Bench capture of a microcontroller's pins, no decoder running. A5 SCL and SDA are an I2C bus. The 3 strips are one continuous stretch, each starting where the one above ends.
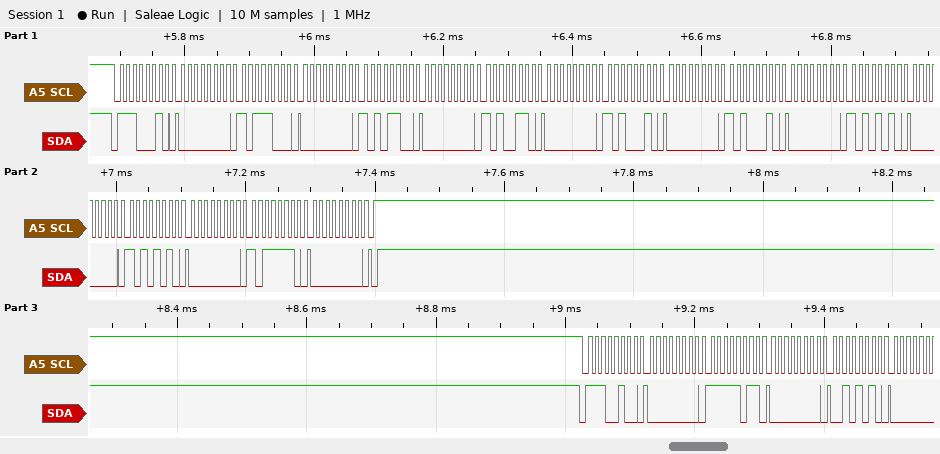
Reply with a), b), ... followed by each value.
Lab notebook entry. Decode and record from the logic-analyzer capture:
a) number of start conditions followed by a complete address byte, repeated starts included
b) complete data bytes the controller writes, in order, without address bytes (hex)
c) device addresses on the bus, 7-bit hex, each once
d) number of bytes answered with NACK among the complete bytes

a) 2
b) 00 B8 00 AC 00 A6 00 A2 00 A2 00 AA 00 AA 00 BE 00 00 FB 00 2A
c) 0x71 0x72
d) 0
